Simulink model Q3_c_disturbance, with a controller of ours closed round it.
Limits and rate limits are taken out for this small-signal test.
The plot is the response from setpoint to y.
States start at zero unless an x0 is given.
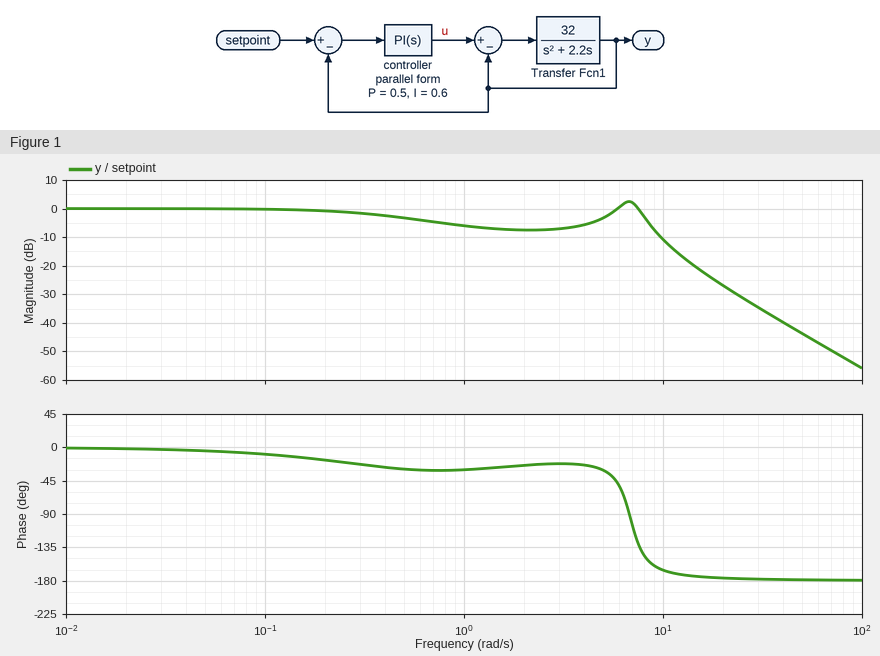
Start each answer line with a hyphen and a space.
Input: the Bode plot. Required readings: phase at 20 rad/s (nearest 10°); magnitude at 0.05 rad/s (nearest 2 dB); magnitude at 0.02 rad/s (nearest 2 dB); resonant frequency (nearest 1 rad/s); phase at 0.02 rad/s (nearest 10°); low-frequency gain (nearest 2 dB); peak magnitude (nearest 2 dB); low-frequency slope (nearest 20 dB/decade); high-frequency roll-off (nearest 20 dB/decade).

- -180°
- 0 dB
- 0 dB
- 7 rad/s
- 0°
- 0 dB
- 2 dB
- 0 dB/decade
- -40 dB/decade
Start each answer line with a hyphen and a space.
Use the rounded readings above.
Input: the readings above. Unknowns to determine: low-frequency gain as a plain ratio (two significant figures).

- 1.0
